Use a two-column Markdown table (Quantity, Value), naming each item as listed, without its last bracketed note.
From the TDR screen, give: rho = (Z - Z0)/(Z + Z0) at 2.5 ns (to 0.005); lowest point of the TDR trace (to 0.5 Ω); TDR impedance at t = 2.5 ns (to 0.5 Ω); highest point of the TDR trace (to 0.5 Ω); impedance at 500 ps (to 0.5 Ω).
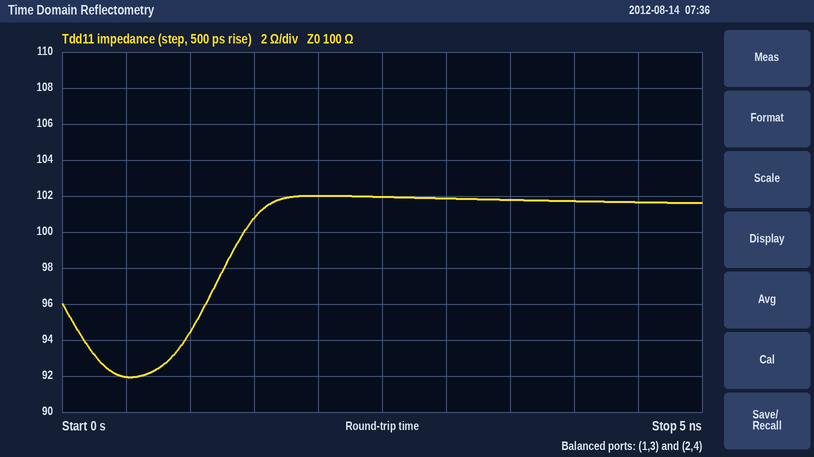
| Quantity | Value |
|---|---|
| rho = (Z - Z0)/(Z + Z0) at 2.5 ns | +0.010 |
| lowest point of the TDR trace | 92.0 Ω |
| TDR impedance at t = 2.5 ns | 102.0 Ω |
| highest point of the TDR trace | 102.0 Ω |
| impedance at 500 ps | 92.0 Ω |
